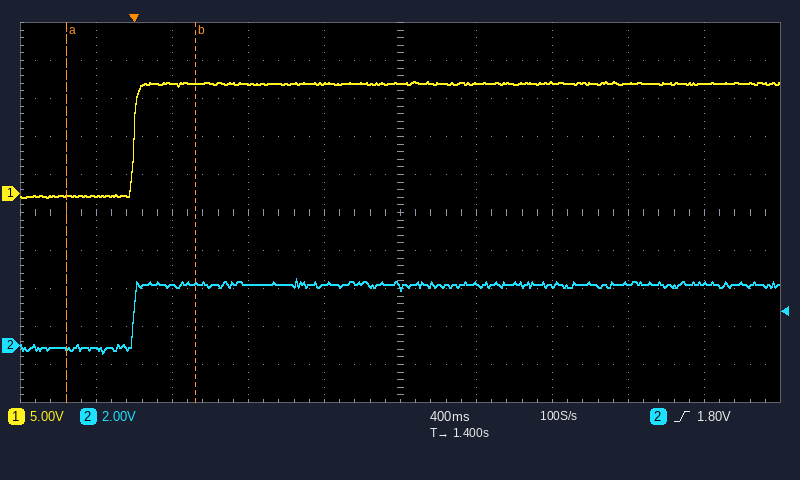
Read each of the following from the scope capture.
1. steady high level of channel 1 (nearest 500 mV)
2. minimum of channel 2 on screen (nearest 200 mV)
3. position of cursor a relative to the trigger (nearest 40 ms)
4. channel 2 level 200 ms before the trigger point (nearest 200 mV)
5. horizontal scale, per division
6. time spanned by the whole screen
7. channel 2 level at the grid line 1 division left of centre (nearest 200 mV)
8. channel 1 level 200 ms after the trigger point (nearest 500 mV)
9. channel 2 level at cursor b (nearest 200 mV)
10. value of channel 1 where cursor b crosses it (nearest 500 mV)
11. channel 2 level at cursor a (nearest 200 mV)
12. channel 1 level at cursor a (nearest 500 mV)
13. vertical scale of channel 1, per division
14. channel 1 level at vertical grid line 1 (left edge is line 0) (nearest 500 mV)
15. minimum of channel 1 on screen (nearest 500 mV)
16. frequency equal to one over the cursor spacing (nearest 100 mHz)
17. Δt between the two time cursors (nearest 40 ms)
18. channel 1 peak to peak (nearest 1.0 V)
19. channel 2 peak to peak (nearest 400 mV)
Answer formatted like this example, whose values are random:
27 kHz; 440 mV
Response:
14.5 V; -400 mV; -360 ms; -200 mV; 400 ms; 4 s; 3.2 V; 14.5 V; 3.2 V; 14.5 V; -200 mV; -500 mV; 5 V; -500 mV; -500 mV; 1.5 Hz; 680 ms; 15.0 V; 4.0 V
